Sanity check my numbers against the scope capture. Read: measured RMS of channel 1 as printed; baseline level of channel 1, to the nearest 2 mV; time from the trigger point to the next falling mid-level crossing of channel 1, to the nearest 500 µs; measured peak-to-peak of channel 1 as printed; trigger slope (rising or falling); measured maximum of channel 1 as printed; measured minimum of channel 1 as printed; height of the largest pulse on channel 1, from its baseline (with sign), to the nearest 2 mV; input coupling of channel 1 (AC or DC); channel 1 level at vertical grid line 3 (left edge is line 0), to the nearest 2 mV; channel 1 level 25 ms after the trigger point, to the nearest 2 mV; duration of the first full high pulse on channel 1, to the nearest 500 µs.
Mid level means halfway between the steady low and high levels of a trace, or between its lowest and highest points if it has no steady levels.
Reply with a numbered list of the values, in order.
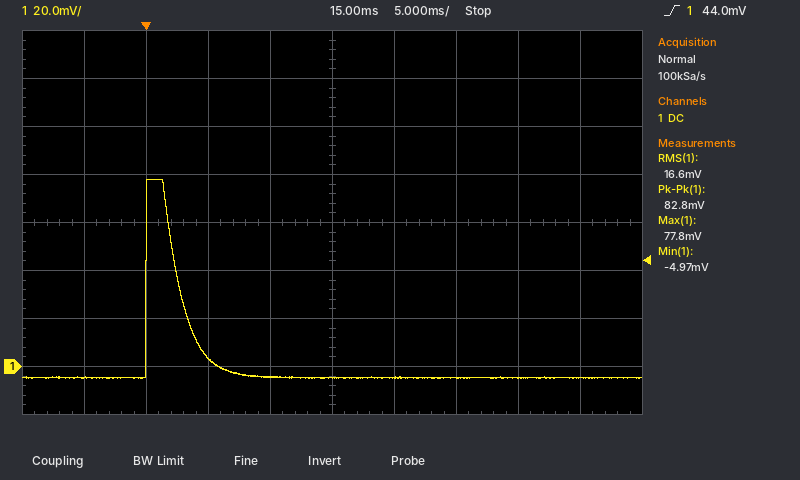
1. 16.6 mV
2. -4 mV
3. 2.5 ms
4. 82.8 mV
5. rising
6. 77.8 mV
7. -4.97 mV
8. +82 mV
9. DC
10. 4 mV
11. -4 mV
12. 2.5 ms
